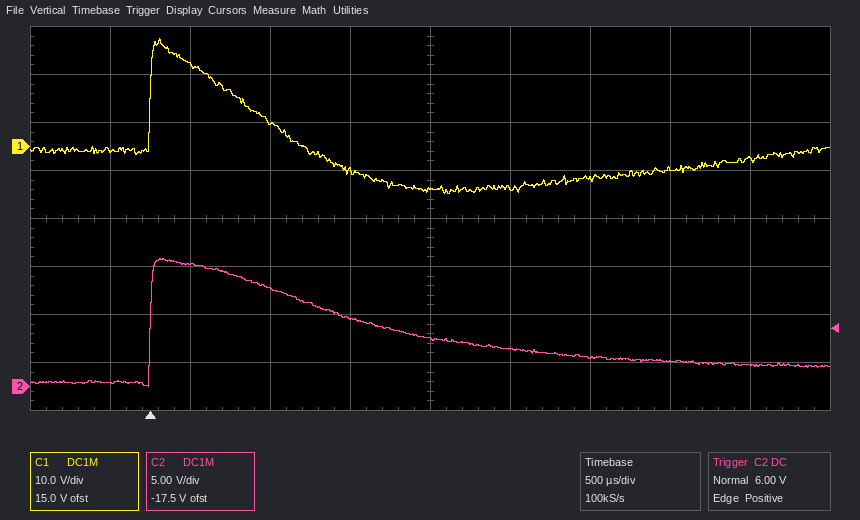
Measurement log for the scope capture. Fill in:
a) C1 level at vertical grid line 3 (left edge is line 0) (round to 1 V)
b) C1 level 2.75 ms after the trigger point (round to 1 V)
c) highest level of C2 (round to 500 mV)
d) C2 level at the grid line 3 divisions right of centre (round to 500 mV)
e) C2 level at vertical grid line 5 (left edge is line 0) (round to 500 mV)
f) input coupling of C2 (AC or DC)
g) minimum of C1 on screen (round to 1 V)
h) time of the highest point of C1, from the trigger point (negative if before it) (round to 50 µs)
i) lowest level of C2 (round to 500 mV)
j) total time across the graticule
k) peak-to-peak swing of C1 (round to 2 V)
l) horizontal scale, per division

5 V
-7 V
13.5 V
2.5 V
5.0 V
DC
-10 V
+50 µs
0.0 V
5 ms
32 V
500 µs
